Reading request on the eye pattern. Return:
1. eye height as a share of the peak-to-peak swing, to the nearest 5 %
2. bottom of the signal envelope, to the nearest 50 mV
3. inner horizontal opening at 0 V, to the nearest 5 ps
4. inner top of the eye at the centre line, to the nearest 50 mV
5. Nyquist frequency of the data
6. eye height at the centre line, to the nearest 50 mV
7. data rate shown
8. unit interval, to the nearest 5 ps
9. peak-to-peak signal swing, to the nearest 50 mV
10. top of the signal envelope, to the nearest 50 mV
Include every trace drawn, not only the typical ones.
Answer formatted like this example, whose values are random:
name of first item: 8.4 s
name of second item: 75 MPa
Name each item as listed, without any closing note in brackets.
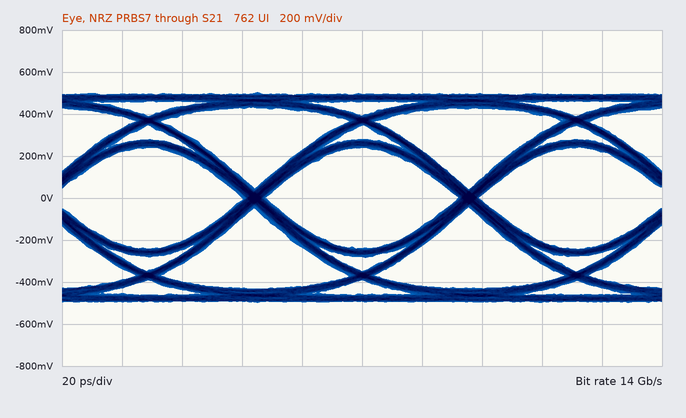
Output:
eye height as a share of the peak-to-peak swing, to the nearest 5 %: 50 %
bottom of the signal envelope, to the nearest 50 mV: -500 mV
inner horizontal opening at 0 V, to the nearest 5 ps: 65 ps
inner top of the eye at the centre line, to the nearest 50 mV: 250 mV
Nyquist frequency of the data: 7 GHz
eye height at the centre line, to the nearest 50 mV: 500 mV
data rate shown: 14 Gb/s
unit interval, to the nearest 5 ps: 70 ps
peak-to-peak signal swing, to the nearest 50 mV: 1.00 V
top of the signal envelope, to the nearest 50 mV: 500 mV
